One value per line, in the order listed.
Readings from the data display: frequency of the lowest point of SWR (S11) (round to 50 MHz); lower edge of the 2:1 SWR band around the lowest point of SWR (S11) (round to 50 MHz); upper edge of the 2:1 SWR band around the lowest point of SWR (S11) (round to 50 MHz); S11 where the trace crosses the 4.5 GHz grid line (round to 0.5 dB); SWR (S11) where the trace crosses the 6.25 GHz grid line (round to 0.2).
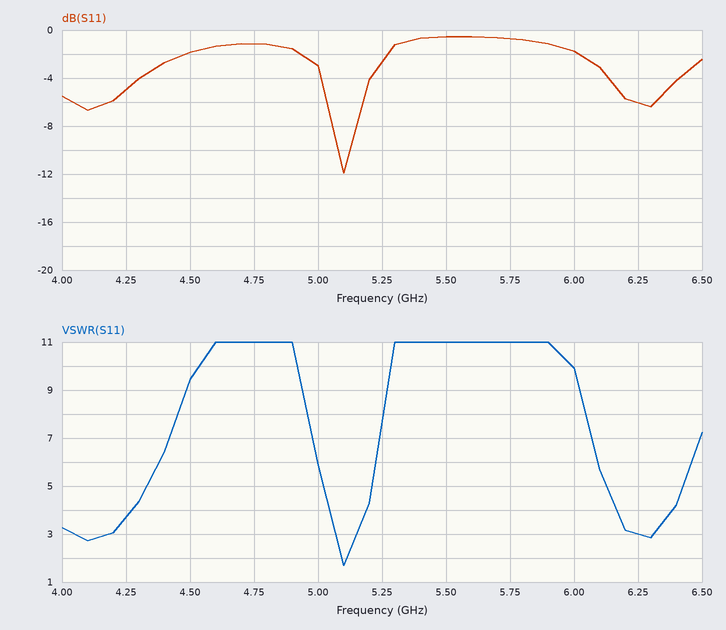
5.10 GHz
5.10 GHz
5.10 GHz
-2.0 dB
3.0
